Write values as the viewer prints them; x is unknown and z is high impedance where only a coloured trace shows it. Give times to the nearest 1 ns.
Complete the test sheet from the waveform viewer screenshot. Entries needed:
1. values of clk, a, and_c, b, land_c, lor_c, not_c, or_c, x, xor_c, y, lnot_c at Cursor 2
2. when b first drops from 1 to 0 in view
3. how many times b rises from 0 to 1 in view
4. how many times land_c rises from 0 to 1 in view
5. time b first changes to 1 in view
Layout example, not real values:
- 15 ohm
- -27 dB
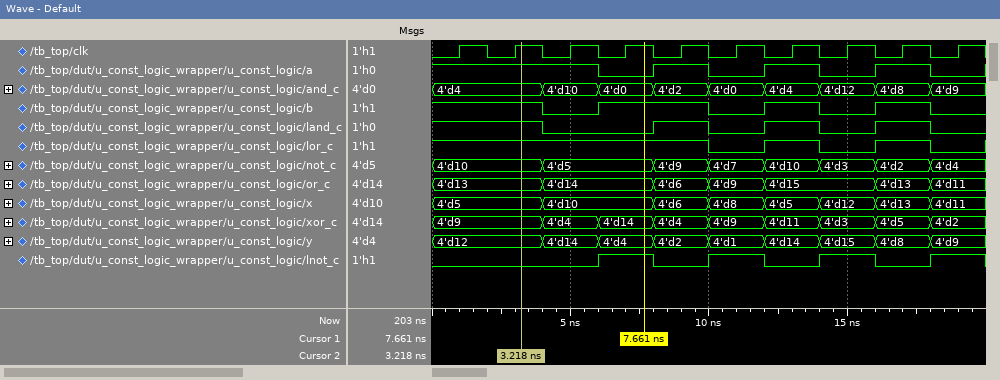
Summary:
- clk=1, a=1, and_c=4'd4, b=1, land_c=1, lor_c=1, not_c=4'd10, or_c=4'd13, x=4'd5, xor_c=4'd9, y=4'd12, lnot_c=0
- 4 ns
- 3
- 3
- 6 ns
